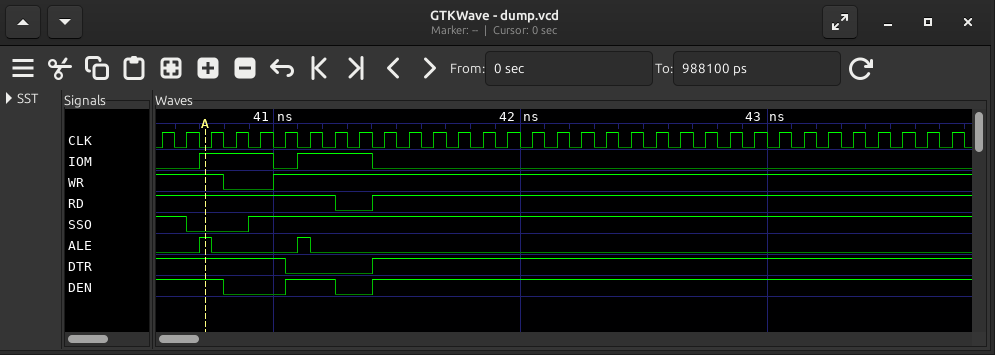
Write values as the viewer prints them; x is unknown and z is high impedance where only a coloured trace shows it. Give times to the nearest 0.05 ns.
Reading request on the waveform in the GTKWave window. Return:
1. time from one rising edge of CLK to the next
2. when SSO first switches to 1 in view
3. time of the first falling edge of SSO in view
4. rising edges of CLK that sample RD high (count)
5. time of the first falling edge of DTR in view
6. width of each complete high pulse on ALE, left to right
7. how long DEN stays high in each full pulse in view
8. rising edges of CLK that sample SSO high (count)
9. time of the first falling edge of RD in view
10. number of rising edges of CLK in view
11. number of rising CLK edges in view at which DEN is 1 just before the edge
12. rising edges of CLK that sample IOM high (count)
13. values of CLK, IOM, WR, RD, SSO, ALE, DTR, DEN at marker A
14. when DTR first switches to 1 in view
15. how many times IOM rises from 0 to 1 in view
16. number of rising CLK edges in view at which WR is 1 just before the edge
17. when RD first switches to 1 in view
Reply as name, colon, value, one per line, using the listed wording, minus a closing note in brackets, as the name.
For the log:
time from one rising edge of CLK to the next: 0.1 ns
when SSO first switches to 1 in view: 40.9 ns
time of the first falling edge of SSO in view: 40.65 ns
rising edges of CLK that sample RD high: 32
time of the first falling edge of DTR in view: 41.05 ns
width of each complete high pulse on ALE, left to right: 0.05 ns, 0.05 ns
how long DEN stays high in each full pulse in view: 0.2 ns
rising edges of CLK that sample SSO high: 31
time of the first falling edge of RD in view: 41.25 ns
number of rising edges of CLK in view: 33
number of rising CLK edges in view at which DEN is 1 just before the edge: 29
rising edges of CLK that sample IOM high: 6
values of CLK, IOM, WR, RD, SSO, ALE, DTR, DEN at marker A: CLK=0, IOM=1, WR=1, RD=1, SSO=0, ALE=1, DTR=1, DEN=1
when DTR first switches to 1 in view: 41.4 ns
how many times IOM rises from 0 to 1 in view: 2
number of rising CLK edges in view at which WR is 1 just before the edge: 31
when RD first switches to 1 in view: 41.4 ns
